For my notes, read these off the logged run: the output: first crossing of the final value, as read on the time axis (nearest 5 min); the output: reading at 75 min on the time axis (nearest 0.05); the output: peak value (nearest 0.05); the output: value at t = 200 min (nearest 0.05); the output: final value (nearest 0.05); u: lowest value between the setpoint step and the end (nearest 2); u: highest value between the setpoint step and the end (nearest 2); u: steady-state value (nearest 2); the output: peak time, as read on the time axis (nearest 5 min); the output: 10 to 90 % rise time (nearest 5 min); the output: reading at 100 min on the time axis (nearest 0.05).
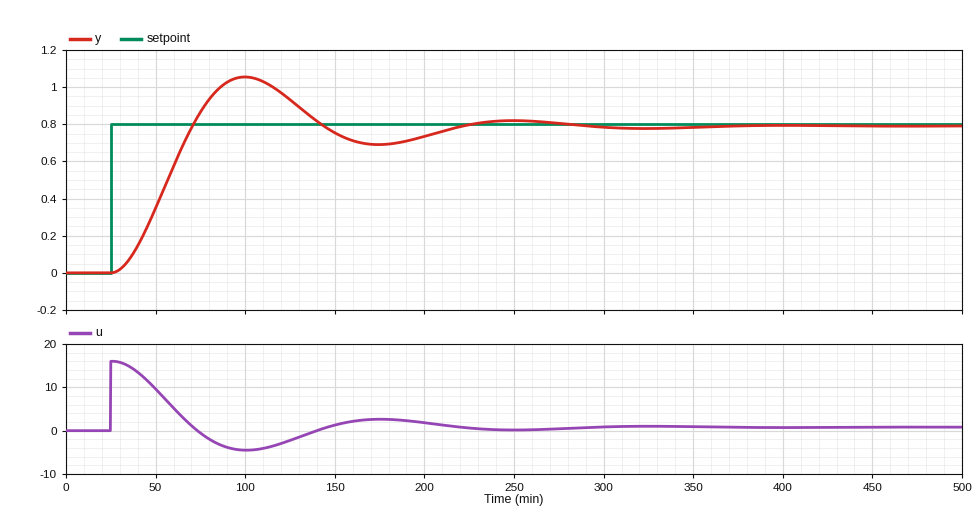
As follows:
70 min
0.85
1.05
0.75
0.80
-4
16
0
100 min
30 min
1.05
